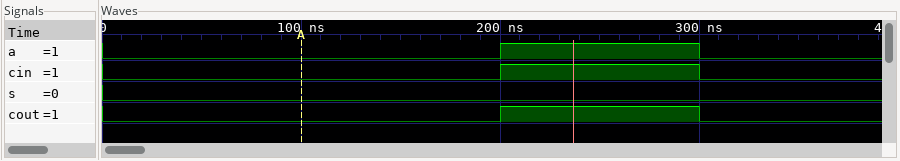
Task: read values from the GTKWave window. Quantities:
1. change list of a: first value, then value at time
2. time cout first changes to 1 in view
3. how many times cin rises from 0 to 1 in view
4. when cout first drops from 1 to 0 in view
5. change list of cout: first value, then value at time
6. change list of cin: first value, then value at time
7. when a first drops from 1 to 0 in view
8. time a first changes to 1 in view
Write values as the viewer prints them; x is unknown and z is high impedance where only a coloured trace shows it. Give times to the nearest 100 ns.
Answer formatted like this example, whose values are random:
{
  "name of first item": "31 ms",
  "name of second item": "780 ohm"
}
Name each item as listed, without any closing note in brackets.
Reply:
{
  "change list of a: first value, then value at time": "0, 1 at 200 ns, 0 at 300 ns",
  "time cout first changes to 1 in view": "200 ns",
  "how many times cin rises from 0 to 1 in view": "1",
  "when cout first drops from 1 to 0 in view": "300 ns",
  "change list of cout: first value, then value at time": "0, 1 at 200 ns, 0 at 300 ns",
  "change list of cin: first value, then value at time": "0, 1 at 200 ns, 0 at 300 ns",
  "when a first drops from 1 to 0 in view": "300 ns",
  "time a first changes to 1 in view": "200 ns"
}
